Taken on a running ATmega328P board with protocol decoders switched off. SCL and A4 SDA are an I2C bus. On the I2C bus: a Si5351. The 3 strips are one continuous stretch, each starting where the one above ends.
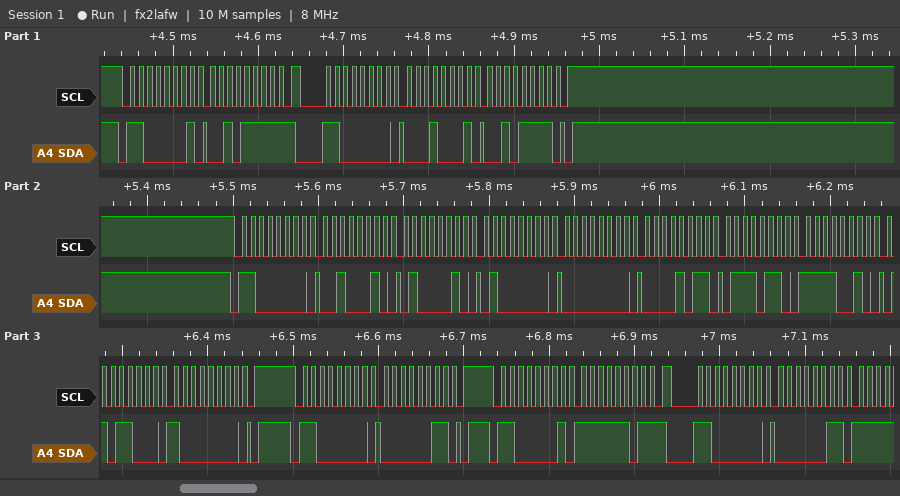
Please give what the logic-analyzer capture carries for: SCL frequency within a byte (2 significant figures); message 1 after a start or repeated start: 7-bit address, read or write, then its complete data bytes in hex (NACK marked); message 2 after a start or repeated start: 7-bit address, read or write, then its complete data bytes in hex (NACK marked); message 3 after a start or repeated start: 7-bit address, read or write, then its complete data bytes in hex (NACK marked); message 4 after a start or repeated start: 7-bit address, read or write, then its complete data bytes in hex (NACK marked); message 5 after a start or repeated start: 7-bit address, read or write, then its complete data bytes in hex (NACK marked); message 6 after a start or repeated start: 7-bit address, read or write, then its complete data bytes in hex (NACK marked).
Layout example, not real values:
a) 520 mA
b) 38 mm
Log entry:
a) 100 kHz
b) 0x60 read: 2F NACK
c) 0x60 write: 11 2F
d) 0x60 write: 22 42 40 00 0B 76 F2 58 80
e) 0x60 write: 03
f) 0x60 read: FD NACK
g) 0x60 write: 03
